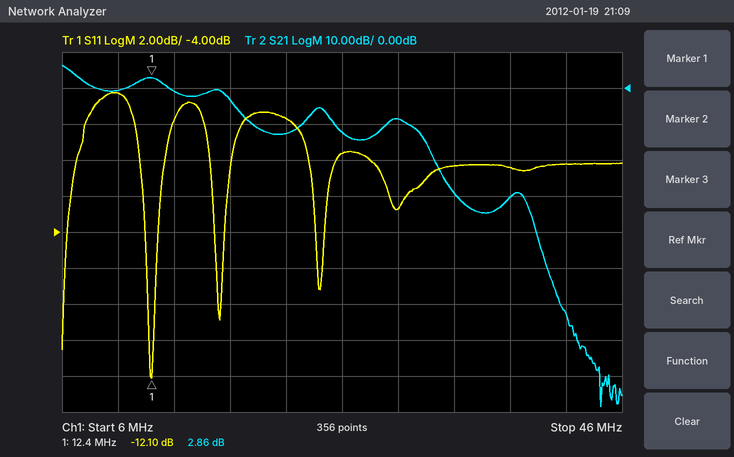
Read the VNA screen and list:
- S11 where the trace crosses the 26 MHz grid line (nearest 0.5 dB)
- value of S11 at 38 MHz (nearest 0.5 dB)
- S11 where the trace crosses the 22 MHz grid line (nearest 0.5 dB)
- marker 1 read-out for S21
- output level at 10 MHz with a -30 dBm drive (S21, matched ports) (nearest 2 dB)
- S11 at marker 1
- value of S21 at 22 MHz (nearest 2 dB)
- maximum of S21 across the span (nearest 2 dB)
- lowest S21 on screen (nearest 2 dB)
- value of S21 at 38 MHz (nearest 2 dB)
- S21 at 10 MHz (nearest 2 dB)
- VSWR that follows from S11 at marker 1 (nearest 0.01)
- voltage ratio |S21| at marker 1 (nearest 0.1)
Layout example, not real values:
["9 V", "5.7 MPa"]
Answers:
["0.5 dB", "-0.5 dB", "2.5 dB", "2.86 dB", "-30 dBm", "-12.10 dB", "-12 dB", "6 dB", "-88 dB", "-30 dB", "0 dB", "1.66", "1.4"]
